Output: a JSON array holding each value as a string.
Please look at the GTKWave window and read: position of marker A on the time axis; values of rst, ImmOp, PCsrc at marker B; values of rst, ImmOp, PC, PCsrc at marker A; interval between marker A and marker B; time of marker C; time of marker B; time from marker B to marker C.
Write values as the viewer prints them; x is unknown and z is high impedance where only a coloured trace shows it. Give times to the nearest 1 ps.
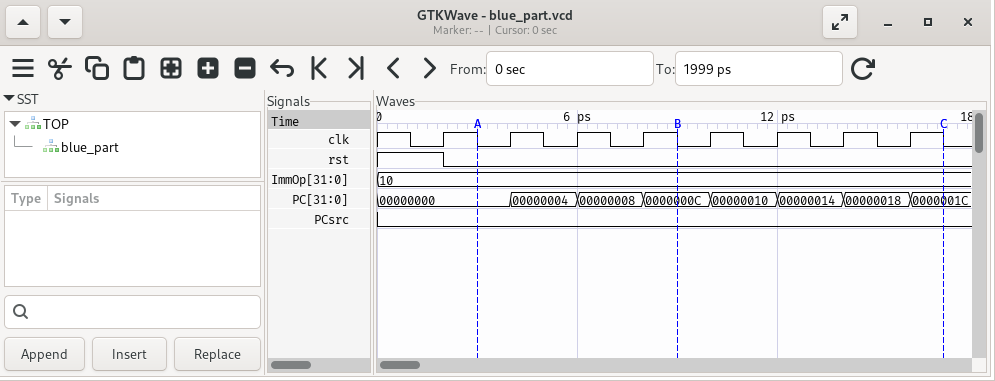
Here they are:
["3 ps", "rst=0, ImmOp=10, PCsrc=0", "rst=0, ImmOp=10, PC=00000000, PCsrc=0", "6 ps", "17 ps", "9 ps", "8 ps"]
